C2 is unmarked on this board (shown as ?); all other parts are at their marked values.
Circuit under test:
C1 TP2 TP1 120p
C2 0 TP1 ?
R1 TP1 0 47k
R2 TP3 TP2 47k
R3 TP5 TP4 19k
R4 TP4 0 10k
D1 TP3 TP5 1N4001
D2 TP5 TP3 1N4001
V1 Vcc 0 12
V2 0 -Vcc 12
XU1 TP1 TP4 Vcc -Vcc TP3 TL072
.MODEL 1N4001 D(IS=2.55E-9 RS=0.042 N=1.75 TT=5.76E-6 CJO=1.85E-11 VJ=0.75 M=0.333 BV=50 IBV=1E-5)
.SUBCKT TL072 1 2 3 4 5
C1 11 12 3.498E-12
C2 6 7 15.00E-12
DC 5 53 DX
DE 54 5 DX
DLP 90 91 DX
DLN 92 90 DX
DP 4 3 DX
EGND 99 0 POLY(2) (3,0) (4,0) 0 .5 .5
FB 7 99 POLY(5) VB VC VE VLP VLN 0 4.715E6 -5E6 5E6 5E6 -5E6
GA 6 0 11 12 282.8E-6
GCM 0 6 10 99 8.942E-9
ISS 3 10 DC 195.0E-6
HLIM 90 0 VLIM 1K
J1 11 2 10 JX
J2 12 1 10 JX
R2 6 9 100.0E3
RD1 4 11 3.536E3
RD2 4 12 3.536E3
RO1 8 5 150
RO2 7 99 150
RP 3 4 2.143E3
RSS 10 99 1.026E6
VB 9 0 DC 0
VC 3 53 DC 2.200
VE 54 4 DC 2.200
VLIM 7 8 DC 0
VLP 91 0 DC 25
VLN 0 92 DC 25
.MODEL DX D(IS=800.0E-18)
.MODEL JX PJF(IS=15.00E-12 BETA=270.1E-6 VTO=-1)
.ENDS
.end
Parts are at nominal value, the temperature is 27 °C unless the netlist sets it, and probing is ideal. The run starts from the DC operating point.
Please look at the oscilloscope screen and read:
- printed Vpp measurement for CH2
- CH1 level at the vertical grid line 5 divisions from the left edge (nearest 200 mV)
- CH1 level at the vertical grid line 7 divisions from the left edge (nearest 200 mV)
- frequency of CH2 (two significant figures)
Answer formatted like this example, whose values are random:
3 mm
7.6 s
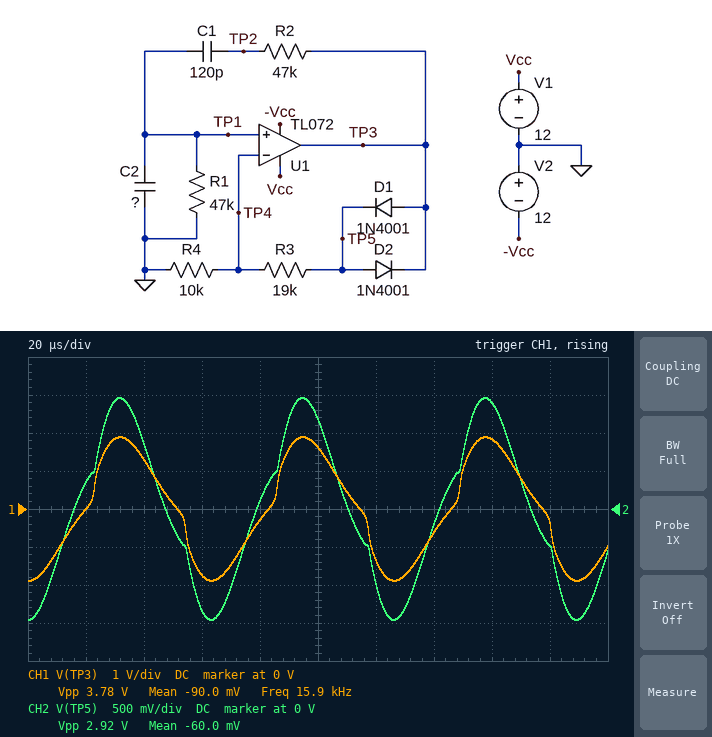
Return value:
2.92 V
1.6 V
-600 mV
16 kHz
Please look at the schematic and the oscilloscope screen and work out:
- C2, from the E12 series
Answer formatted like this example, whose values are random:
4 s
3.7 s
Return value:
220 pF
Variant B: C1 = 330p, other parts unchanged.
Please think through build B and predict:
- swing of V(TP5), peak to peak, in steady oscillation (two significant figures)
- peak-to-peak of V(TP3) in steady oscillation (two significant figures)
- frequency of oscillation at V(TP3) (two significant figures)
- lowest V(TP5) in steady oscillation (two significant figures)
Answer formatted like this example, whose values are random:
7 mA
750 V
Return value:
20 V
21 V
11 kHz
-10 V
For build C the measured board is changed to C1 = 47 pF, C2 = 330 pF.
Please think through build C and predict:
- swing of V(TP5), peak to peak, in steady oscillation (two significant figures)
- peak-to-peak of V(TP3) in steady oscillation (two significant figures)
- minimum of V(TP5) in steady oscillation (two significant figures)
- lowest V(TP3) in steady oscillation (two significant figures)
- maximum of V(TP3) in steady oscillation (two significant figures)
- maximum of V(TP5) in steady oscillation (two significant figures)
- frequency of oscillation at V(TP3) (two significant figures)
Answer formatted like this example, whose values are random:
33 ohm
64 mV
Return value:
360 mV
1.0 V
-180 mV
-500 mV
500 mV
180 mV
9.9 kHz
